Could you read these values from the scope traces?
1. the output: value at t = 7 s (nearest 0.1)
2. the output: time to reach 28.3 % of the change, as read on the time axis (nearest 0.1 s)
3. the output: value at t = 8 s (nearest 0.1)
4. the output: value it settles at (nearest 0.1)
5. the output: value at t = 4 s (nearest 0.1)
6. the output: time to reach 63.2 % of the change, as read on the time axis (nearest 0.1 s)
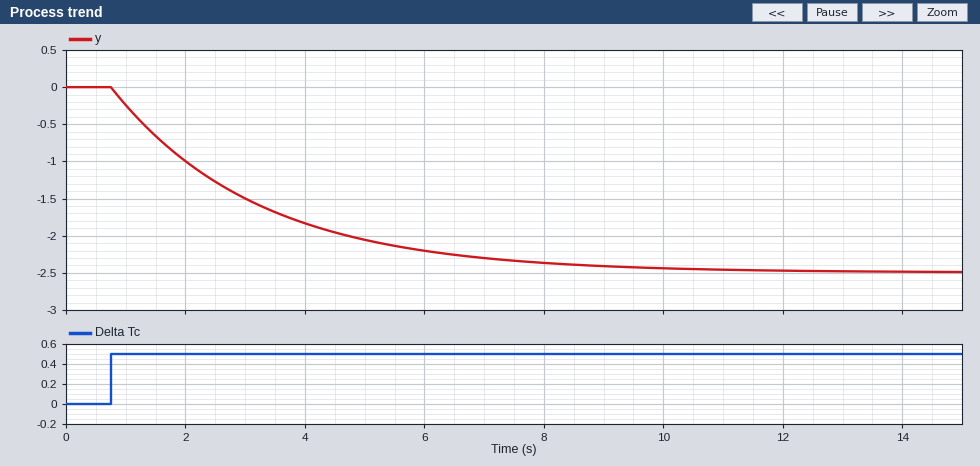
-2.3
1.6 s
-2.4
-2.5
-1.8
3.2 s
